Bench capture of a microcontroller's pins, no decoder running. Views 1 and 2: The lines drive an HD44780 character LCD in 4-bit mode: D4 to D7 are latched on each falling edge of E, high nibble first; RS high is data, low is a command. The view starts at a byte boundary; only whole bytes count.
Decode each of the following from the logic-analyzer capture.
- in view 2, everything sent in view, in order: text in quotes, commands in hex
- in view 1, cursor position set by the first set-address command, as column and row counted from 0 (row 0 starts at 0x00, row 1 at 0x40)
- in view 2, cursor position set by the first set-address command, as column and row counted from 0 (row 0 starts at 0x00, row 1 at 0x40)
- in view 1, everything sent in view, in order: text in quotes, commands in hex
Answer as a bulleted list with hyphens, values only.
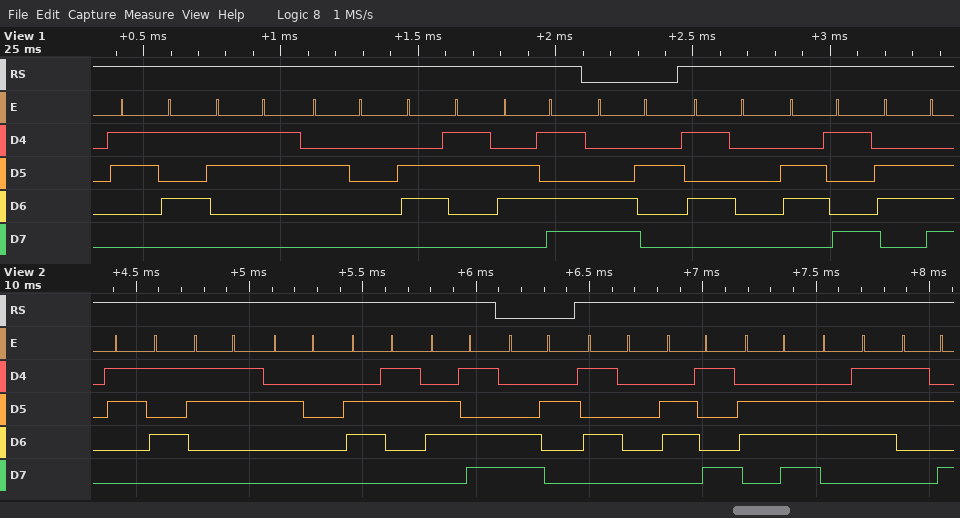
- "53 cm" 0xC2 "Ping:"
- column 2, row 1
- column 2, row 1
- "53 cm" 0xC2 "Pin"
